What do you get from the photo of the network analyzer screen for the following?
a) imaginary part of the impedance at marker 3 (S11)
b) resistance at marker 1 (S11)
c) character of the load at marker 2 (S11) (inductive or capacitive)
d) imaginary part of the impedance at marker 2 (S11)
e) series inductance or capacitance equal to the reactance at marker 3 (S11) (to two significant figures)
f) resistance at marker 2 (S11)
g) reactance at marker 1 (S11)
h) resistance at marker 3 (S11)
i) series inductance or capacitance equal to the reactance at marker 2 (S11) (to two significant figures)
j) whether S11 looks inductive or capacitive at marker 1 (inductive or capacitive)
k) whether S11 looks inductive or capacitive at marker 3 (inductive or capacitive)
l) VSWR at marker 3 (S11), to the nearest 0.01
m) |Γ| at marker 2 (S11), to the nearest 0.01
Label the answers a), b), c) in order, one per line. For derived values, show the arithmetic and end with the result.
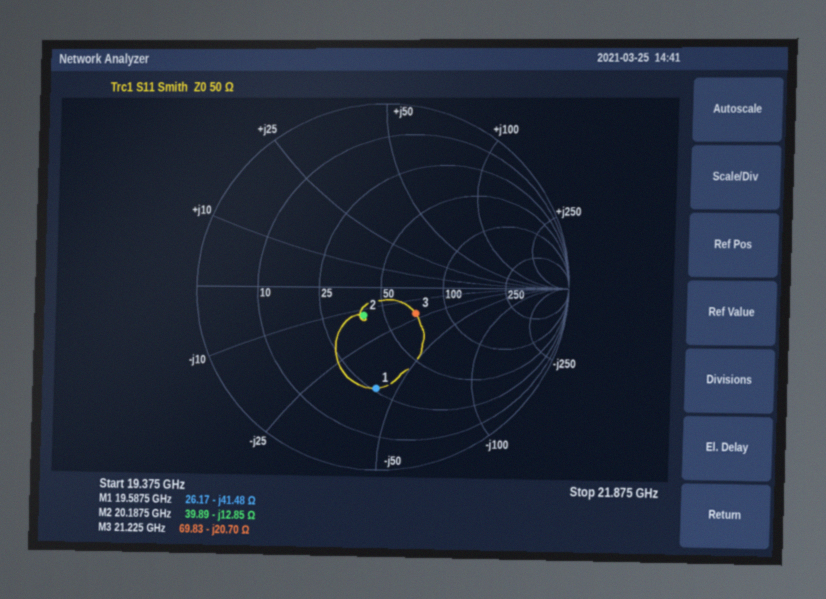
a) -20.70 Ω
b) 26.17 Ω
c) capacitive
d) -12.85 Ω
e) C = 1/(2π × 21.225 GHz × 20.7 Ω) ≈ 362 fF, so 360 fF to two significant figures
f) 39.89 Ω
g) -41.48 Ω
h) 69.83 Ω
i) C = 1/(2π × 20.1875 GHz × 12.85 Ω) ≈ 614 fF, so 610 fF to two significant figures
j) capacitive
k) capacitive
l) 1.62
m) 0.18
